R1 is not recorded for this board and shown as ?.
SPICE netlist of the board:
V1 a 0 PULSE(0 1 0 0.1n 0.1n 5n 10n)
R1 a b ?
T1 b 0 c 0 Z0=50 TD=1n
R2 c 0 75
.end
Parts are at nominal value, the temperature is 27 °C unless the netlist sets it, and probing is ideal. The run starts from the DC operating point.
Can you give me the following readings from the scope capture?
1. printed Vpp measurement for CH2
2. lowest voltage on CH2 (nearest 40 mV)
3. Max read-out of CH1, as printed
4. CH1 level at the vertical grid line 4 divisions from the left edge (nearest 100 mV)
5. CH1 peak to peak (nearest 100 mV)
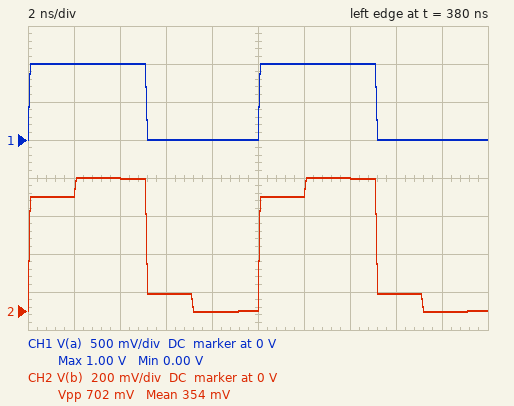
702 mV
0 V
1.00 V
0 V
1.0 V
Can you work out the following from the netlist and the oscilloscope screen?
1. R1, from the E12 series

33 Ω
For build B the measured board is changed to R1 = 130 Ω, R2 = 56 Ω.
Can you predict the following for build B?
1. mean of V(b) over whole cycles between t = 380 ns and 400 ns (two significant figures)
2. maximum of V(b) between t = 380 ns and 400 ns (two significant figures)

150 mV
300 mV
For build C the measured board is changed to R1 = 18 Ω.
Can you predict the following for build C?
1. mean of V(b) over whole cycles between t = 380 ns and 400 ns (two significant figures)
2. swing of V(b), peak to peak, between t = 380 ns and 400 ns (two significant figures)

410 mV
820 mV
